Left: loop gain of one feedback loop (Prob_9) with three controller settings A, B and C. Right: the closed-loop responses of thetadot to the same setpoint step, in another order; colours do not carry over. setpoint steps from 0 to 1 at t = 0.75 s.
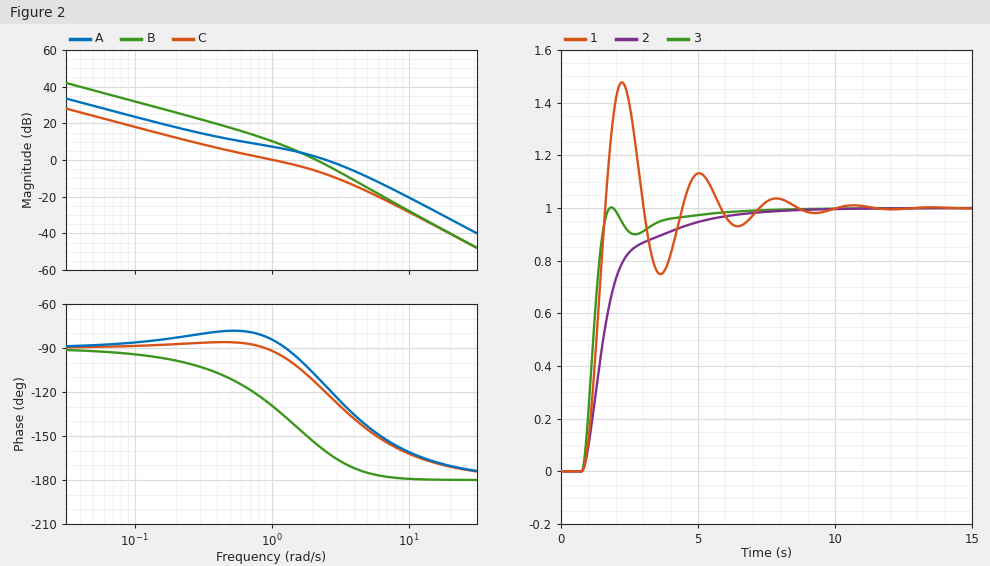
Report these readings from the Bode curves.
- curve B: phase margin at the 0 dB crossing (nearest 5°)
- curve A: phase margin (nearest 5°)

25°
65°
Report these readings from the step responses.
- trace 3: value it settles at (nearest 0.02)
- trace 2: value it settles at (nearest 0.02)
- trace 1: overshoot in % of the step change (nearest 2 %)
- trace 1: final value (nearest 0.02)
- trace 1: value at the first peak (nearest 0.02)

1.00
1.00
48 %
1.00
1.48
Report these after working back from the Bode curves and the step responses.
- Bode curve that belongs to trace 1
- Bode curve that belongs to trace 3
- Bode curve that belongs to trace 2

B
A
C
